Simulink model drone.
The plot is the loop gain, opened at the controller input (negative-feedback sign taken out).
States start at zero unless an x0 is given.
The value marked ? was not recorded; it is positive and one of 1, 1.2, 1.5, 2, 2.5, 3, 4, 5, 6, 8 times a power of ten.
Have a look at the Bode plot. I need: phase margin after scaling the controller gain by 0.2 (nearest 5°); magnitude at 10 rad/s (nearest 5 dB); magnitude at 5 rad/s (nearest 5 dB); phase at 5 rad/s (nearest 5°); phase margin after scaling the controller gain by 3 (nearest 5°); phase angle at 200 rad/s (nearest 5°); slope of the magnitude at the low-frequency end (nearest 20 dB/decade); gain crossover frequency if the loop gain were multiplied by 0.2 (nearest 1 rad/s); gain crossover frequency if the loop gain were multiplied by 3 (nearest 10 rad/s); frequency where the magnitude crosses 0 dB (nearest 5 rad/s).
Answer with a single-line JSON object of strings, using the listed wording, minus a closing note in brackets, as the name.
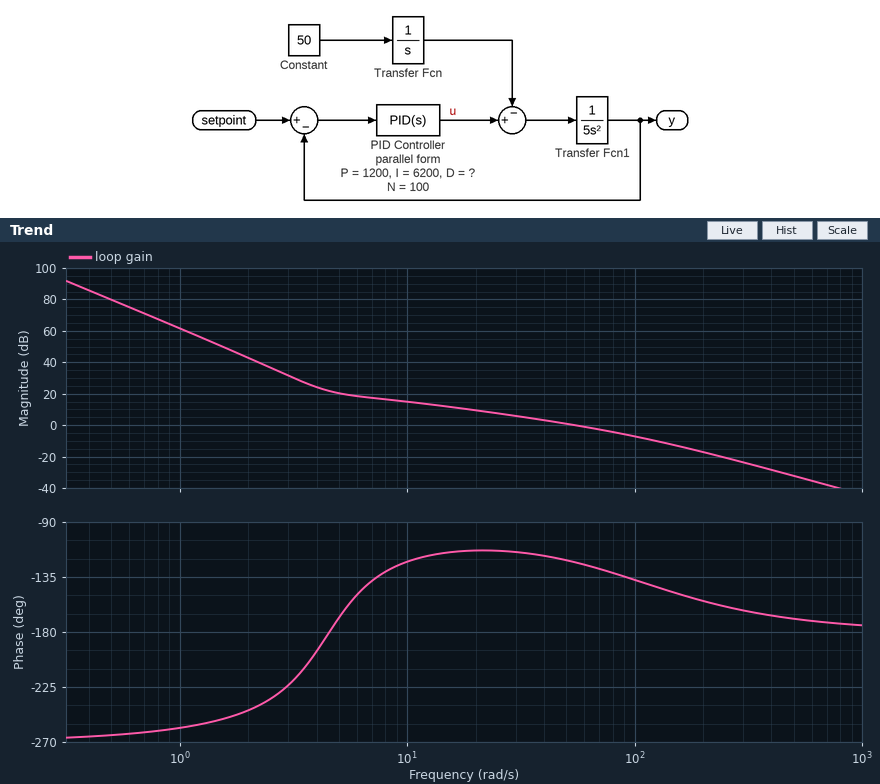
{"phase margin after scaling the controller gain by 0.2": "60°", "magnitude at 10 rad/s": "15 dB", "magnitude at 5 rad/s": "20 dB", "phase at 5 rad/s": "-170°", "phase margin after scaling the controller gain by 3": "40°", "phase angle at 200 rad/s": "-155°", "slope of the magnitude at the low-frequency end": "-60 dB/decade", "gain crossover frequency if the loop gain were multiplied by 0.2": "11 rad/s", "gain crossover frequency if the loop gain were multiplied by 3": "120 rad/s", "frequency where the magnitude crosses 0 dB": "55 rad/s"}
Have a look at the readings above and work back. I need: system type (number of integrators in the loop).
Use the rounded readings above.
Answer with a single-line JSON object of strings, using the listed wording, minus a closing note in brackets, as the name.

{"system type": "3"}
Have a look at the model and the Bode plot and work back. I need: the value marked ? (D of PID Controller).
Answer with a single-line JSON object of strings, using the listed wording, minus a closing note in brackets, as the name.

{"the value marked ?": "300"}
